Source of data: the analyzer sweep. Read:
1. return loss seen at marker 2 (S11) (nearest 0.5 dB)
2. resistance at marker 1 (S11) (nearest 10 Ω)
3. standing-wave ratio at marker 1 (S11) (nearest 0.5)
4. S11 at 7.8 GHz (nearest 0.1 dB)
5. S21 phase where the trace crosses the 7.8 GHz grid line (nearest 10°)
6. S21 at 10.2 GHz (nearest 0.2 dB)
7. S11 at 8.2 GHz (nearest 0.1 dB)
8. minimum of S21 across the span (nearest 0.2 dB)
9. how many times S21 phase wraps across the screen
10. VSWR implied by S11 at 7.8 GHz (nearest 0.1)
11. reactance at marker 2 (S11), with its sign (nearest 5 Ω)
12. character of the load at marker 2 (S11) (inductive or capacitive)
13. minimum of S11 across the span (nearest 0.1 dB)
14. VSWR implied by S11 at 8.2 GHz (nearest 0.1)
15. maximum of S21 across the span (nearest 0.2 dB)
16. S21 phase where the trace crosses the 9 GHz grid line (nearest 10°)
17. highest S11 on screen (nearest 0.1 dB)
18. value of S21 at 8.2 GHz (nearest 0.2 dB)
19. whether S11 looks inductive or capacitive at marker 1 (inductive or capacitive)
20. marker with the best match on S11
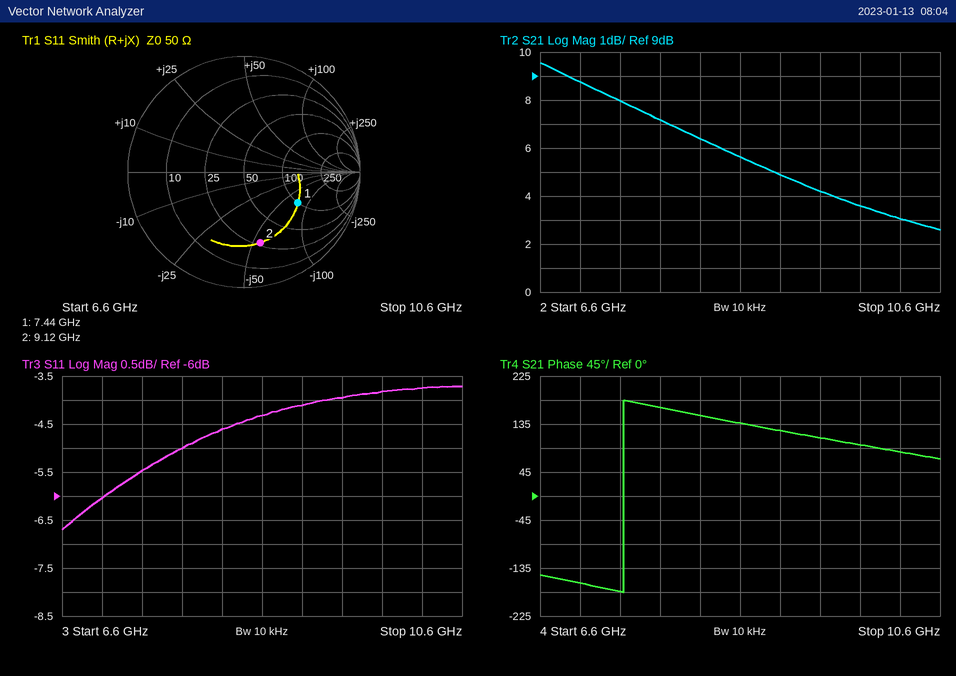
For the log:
4.0 dB
100 Ω
3.5
-5.0 dB
170°
3.0 dB
-4.6 dB
2.6 dB
1
3.6
-55 Ω
capacitive
-6.7 dB
3.9
9.6 dB
120°
-3.7 dB
6.4 dB
capacitive
marker 1
